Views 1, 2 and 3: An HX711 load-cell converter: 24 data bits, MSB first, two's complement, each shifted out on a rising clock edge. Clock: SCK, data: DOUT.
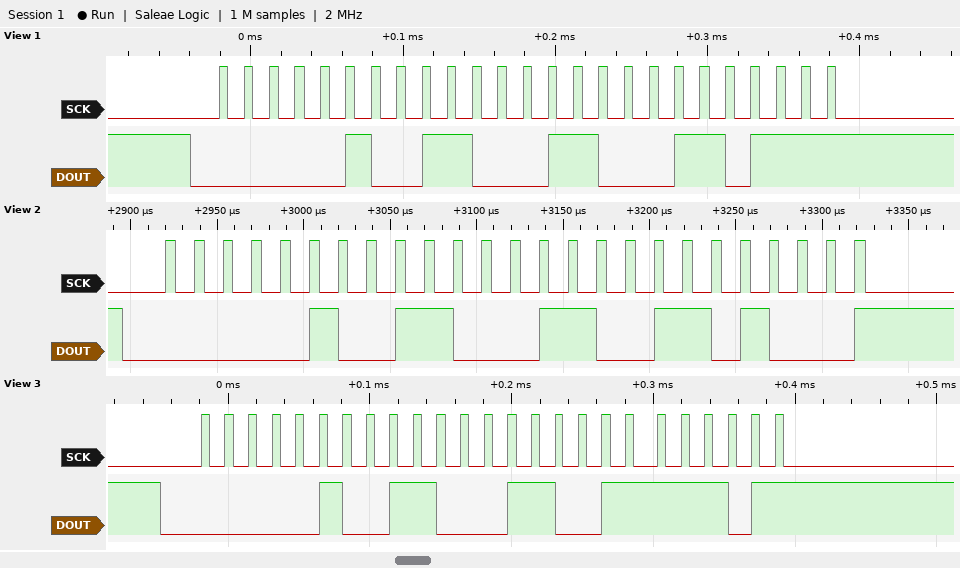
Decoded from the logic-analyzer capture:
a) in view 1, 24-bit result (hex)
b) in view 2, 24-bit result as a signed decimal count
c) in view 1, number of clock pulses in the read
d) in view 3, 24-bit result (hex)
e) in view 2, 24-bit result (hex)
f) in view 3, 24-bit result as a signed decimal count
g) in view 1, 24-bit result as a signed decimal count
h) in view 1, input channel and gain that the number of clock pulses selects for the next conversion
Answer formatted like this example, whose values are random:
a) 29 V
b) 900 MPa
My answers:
a) 0x04C637
b) 312936
c) 25
d) 0x04C67D
e) 0x04C668
f) 312957
g) 312887
h) channel A, gain 128
